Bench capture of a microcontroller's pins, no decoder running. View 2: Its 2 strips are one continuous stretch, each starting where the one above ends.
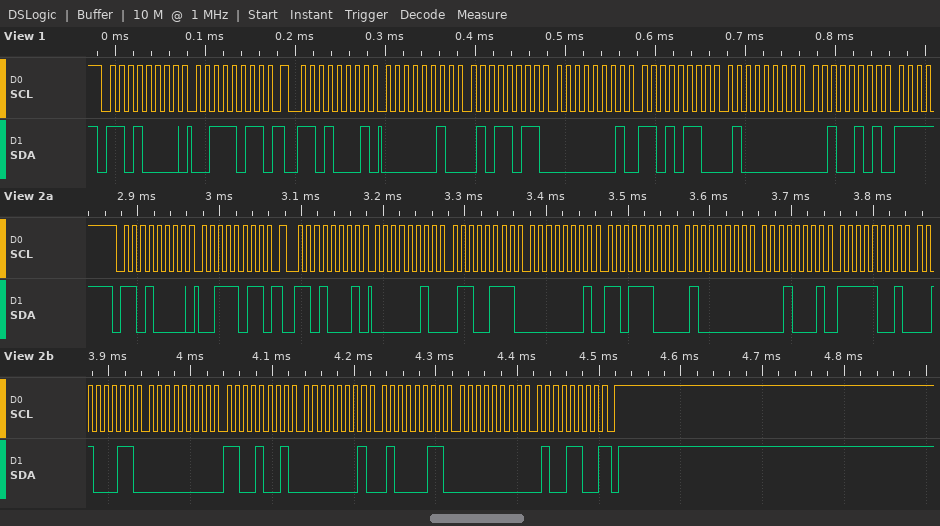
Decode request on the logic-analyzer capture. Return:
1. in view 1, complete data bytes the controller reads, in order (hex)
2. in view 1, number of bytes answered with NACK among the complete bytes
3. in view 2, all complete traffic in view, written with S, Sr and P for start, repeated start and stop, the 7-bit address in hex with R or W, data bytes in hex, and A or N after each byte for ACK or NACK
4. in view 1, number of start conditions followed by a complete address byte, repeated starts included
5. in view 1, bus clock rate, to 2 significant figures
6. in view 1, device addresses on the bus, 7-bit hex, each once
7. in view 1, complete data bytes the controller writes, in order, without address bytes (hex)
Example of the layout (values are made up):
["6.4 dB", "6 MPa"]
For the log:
["02 5B 01 D6 40 25", "0", "S 68W A 3B A Sr 68R A 02 A 67 A 01 A DC A 40 A 11 A F9 A 23 A 00 A C9 A 01 A 43 A 00 A 4C N P", "2", "100 kHz", "0x68", "3B"]
